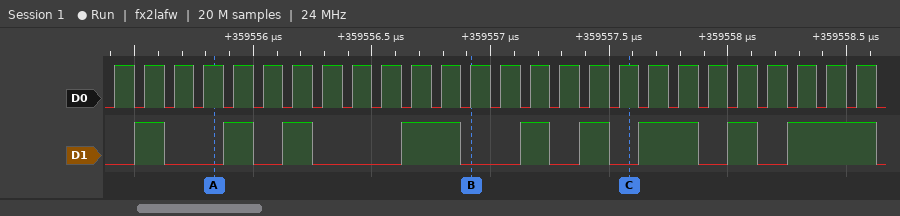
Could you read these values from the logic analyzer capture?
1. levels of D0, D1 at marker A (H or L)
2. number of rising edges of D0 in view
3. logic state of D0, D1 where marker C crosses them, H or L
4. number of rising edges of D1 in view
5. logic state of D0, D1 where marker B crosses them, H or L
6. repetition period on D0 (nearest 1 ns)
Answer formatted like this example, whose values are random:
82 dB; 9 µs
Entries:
D0=H, D1=L; 26; D0=H, D1=L; 9; D0=H, D1=L; 125 ns
